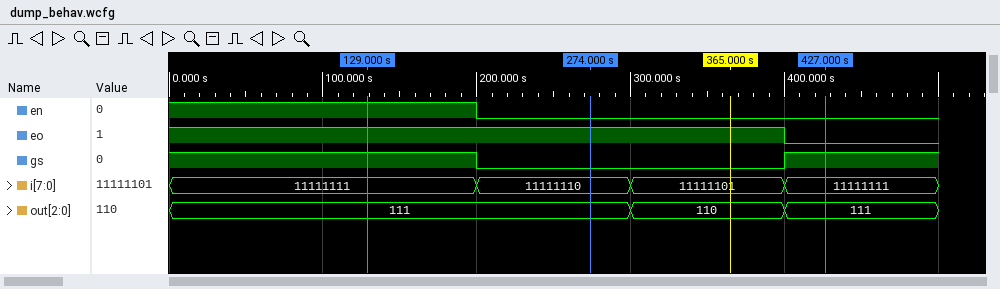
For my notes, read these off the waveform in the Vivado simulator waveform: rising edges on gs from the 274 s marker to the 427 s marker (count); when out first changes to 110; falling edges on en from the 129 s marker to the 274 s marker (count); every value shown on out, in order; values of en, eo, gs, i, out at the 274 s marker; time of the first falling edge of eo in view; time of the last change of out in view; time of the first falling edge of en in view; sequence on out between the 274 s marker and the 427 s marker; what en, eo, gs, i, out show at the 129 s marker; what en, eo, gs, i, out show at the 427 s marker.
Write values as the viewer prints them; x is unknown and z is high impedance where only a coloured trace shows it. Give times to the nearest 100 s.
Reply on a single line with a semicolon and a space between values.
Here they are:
1; 300 s; 1; 111, 110, 111; en=0, eo=1, gs=0, i=11111110, out=111; 400 s; 400 s; 200 s; 111, 110, 111; en=1, eo=1, gs=1, i=11111111, out=111; en=0, eo=0, gs=1, i=11111111, out=111
